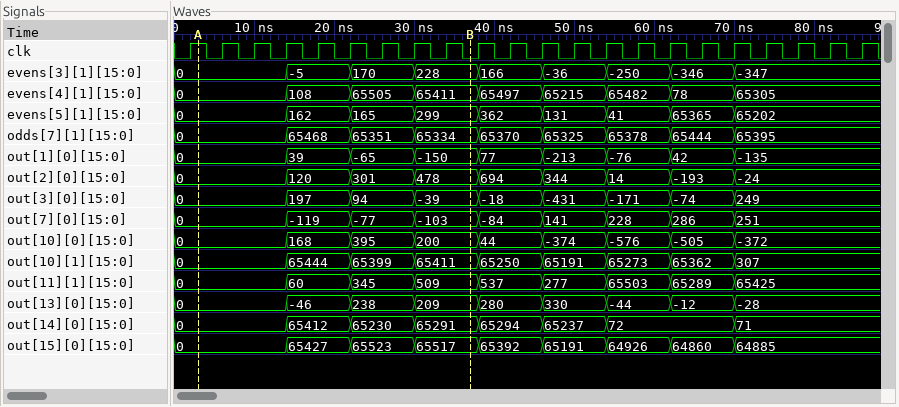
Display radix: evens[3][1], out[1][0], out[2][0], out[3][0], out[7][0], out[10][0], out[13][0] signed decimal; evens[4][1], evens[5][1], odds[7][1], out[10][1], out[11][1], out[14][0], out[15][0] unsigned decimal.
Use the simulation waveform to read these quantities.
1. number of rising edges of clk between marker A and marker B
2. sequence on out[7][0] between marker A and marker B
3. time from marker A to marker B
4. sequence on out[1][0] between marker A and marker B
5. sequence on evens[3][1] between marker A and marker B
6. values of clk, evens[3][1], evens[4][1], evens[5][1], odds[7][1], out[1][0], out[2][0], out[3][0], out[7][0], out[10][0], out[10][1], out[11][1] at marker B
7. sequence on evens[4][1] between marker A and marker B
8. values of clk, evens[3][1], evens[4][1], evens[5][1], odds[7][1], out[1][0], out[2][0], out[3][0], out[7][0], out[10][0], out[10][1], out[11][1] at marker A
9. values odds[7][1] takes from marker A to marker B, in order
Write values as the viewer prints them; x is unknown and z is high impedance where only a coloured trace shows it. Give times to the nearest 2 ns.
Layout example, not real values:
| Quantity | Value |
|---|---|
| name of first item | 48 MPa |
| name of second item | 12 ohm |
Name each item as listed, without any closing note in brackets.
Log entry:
| Quantity | Value |
|---|---|
| number of rising edges of clk between marker A and marker B | 8 |
| sequence on out[7][0] between marker A and marker B | 0, -119, -77, -103 |
| time from marker A to marker B | 34 ns |
| sequence on out[1][0] between marker A and marker B | 0, 39, -65, -150 |
| sequence on evens[3][1] between marker A and marker B | 0, -5, 170, 228 |
| values of clk, evens[3][1], evens[4][1], evens[5][1], odds[7][1], out[1][0], out[2][0], out[3][0], out[7][0], out[10][0], out[10][1], out[11][1] at marker B | clk=0, evens[3][1]=228, evens[4][1]=65411, evens[5][1]=299, odds[7][1]=65334, out[1][0]=-150, out[2][0]=478, out[3][0]=-39, out[7][0]=-103, out[10][0]=200, out[10][1]=65411, out[11][1]=509 |
| sequence on evens[4][1] between marker A and marker B | 0, 108, 65505, 65411 |
| values of clk, evens[3][1], evens[4][1], evens[5][1], odds[7][1], out[1][0], out[2][0], out[3][0], out[7][0], out[10][0], out[10][1], out[11][1] at marker A | clk=1, evens[3][1]=0, evens[4][1]=0, evens[5][1]=0, odds[7][1]=0, out[1][0]=0, out[2][0]=0, out[3][0]=0, out[7][0]=0, out[10][0]=0, out[10][1]=0, out[11][1]=0 |
| values odds[7][1] takes from marker A to marker B, in order | 0, 65468, 65351, 65334 |
